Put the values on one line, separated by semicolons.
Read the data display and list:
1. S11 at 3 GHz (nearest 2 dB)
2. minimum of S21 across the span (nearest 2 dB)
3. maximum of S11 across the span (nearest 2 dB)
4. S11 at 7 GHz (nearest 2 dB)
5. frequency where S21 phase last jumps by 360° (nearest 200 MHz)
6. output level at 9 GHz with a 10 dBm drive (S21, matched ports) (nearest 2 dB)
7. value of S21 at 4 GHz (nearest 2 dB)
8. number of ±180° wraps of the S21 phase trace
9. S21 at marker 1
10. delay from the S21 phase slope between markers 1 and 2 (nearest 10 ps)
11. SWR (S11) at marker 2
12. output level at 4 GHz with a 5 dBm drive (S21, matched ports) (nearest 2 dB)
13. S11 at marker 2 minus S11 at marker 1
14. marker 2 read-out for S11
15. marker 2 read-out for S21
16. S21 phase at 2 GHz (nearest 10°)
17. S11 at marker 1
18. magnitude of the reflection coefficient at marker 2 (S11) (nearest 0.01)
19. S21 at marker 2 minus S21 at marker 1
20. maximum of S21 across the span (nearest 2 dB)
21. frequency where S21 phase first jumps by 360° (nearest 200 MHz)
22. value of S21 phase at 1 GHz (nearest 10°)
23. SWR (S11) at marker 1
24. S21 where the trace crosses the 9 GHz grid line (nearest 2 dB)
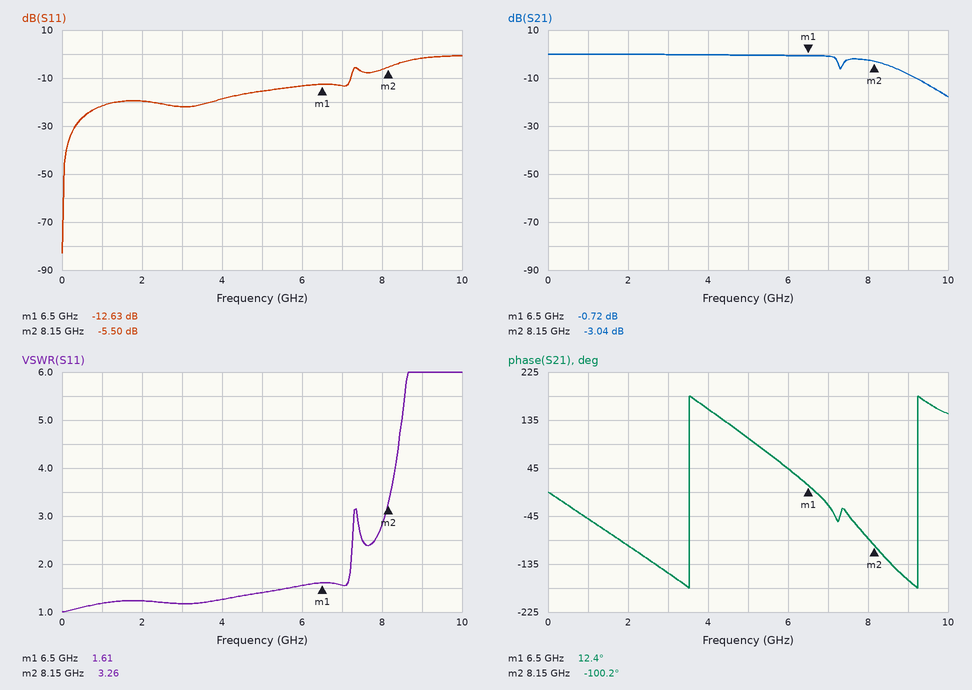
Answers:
-22 dB; -18 dB; 0 dB; -14 dB; 9.2 GHz; 2 dBm; 0 dB; 2; -0.72 dB; 190 ps; 3.26; 4 dBm; 7.13 dB; -5.50 dB; -3.04 dB; -100°; -12.63 dB; 0.53; -2.32 dB; 0 dB; 3.6 GHz; -50°; 1.61; -8 dB
